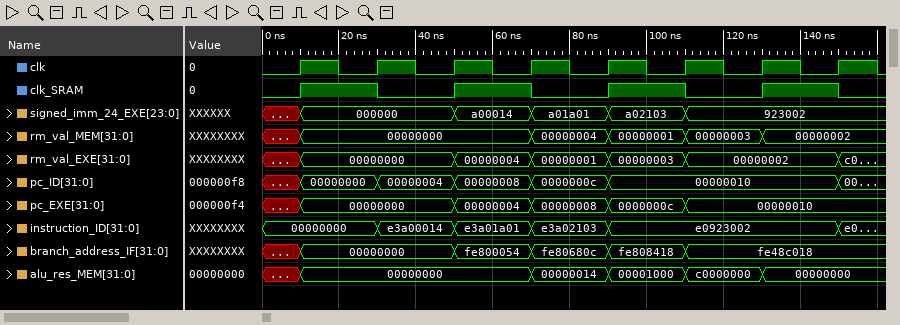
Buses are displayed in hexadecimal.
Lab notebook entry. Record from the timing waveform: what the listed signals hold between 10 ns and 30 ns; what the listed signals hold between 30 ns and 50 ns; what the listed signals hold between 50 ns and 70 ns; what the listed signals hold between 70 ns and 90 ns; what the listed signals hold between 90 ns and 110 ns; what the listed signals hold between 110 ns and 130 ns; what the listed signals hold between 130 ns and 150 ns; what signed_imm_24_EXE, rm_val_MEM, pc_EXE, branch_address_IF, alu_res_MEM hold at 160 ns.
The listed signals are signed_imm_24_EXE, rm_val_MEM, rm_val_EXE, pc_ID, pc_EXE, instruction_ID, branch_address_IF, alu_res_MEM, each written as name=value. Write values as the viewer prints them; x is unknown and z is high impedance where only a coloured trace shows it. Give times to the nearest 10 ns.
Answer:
signed_imm_24_EXE=000000, rm_val_MEM=00000000, rm_val_EXE=00000000, pc_ID=00000000, pc_EXE=00000000, instruction_ID=00000000, branch_address_IF=00000000, alu_res_MEM=00000000
signed_imm_24_EXE=000000, rm_val_MEM=00000000, rm_val_EXE=00000000, pc_ID=00000004, pc_EXE=00000000, instruction_ID=e3a00014, branch_address_IF=00000000, alu_res_MEM=00000000
signed_imm_24_EXE=a00014, rm_val_MEM=00000000, rm_val_EXE=00000004, pc_ID=00000008, pc_EXE=00000004, instruction_ID=e3a01a01, branch_address_IF=fe800054, alu_res_MEM=00000000
signed_imm_24_EXE=a01a01, rm_val_MEM=00000004, rm_val_EXE=00000001, pc_ID=0000000c, pc_EXE=00000008, instruction_ID=e3a02103, branch_address_IF=fe80680c, alu_res_MEM=00000014
signed_imm_24_EXE=a02103, rm_val_MEM=00000001, rm_val_EXE=00000003, pc_ID=00000010, pc_EXE=0000000c, instruction_ID=e0923002, branch_address_IF=fe808418, alu_res_MEM=00001000
signed_imm_24_EXE=923002, rm_val_MEM=00000003, rm_val_EXE=00000002, pc_ID=00000010, pc_EXE=00000010, instruction_ID=e0923002, branch_address_IF=fe48c018, alu_res_MEM=c0000000
signed_imm_24_EXE=923002, rm_val_MEM=00000002, rm_val_EXE=00000002, pc_ID=00000010, pc_EXE=00000010, instruction_ID=e0923002, branch_address_IF=fe48c018, alu_res_MEM=00000000
signed_imm_24_EXE=923002, rm_val_MEM=00000002, pc_EXE=00000010, branch_address_IF=fe48c018, alu_res_MEM=00000000
